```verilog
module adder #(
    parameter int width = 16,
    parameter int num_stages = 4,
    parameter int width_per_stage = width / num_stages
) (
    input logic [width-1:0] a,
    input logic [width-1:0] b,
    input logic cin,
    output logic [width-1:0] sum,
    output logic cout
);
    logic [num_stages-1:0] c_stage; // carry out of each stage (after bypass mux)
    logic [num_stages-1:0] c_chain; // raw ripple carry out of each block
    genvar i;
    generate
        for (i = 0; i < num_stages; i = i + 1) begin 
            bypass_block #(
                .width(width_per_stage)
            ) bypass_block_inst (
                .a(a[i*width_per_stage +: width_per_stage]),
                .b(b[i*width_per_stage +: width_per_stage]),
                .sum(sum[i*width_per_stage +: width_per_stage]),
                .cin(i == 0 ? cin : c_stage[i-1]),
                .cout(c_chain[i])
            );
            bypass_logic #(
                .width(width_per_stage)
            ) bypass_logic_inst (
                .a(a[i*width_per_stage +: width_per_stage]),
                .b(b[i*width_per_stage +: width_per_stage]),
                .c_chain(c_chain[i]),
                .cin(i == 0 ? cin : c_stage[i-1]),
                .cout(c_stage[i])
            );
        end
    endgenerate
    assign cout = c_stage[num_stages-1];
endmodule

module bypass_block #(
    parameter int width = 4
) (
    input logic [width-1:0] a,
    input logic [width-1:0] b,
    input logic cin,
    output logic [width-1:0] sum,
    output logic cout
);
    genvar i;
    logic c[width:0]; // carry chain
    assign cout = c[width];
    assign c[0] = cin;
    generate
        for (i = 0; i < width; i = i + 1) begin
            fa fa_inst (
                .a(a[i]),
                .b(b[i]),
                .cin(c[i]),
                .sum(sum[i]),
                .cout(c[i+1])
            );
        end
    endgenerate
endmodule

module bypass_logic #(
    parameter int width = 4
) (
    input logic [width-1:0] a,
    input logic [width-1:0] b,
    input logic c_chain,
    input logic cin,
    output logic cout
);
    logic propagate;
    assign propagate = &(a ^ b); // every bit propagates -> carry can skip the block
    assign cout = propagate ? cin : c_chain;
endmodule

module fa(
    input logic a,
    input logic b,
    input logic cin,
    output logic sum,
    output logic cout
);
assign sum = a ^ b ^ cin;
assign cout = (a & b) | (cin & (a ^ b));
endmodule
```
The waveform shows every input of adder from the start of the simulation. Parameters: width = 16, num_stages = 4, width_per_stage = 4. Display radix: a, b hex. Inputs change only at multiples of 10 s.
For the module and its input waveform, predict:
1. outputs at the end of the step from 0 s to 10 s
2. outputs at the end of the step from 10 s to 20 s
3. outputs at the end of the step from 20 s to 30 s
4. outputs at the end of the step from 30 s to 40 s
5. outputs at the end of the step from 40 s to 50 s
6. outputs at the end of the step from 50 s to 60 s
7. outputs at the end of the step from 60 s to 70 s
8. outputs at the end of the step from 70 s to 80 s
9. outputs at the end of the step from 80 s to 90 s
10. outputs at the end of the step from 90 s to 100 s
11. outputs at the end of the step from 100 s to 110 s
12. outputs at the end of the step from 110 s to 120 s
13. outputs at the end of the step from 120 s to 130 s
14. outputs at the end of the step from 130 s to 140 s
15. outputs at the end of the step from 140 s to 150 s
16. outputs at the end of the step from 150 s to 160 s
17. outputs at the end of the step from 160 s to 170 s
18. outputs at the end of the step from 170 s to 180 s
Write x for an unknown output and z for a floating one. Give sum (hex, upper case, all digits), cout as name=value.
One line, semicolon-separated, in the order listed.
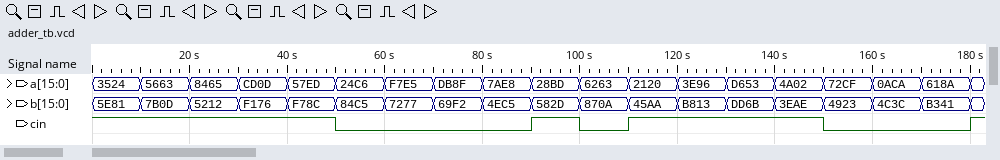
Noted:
sum=93A6, cout=0; sum=D171, cout=0; sum=D678, cout=0; sum=BE84, cout=1; sum=4F7A, cout=1; sum=A98B, cout=0; sum=6A5C, cout=1; sum=4581, cout=1; sum=C9AD, cout=0; sum=80EB, cout=0; sum=E96D, cout=0; sum=66CB, cout=0; sum=F6AA, cout=0; sum=B3BF, cout=1; sum=88B1, cout=0; sum=BBF2, cout=0; sum=5706, cout=0; sum=14CB, cout=1
